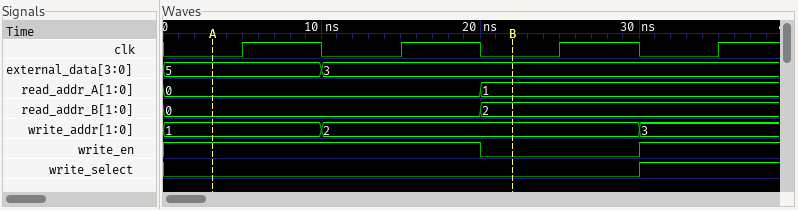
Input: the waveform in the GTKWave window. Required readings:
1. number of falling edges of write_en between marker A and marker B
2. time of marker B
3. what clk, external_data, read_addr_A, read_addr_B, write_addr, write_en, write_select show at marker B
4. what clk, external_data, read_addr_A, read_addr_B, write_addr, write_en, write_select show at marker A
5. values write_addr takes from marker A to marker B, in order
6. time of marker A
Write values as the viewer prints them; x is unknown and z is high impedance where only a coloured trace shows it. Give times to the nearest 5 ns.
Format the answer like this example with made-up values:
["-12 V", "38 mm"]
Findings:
["1", "20 ns", "clk=0, external_data=3, read_addr_A=1, read_addr_B=2, write_addr=2, write_en=0, write_select=0", "clk=0, external_data=5, read_addr_A=0, read_addr_B=0, write_addr=1, write_en=1, write_select=0", "1, 2", "5 ns"]
